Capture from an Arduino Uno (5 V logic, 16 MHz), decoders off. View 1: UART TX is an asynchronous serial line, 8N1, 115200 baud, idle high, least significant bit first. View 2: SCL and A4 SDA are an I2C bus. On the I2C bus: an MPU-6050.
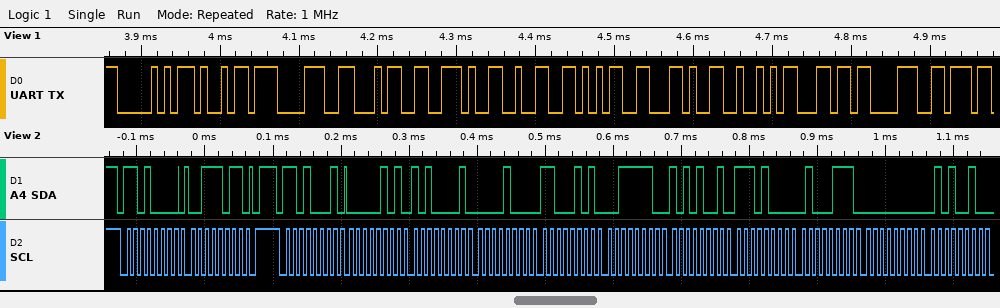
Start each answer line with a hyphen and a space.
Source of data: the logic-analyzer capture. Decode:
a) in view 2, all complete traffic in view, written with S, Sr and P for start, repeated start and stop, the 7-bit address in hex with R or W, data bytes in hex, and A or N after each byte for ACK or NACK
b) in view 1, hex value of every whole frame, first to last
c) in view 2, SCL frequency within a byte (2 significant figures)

- S 68W A 3B A P S 68R A 05 A A1 A 08 A C5 A 3E A A9 A E8 A 47 A 00 A 52 A
- 50 69 38 34 2E 32 35 2C 52 6C 38
- 100 kHz
